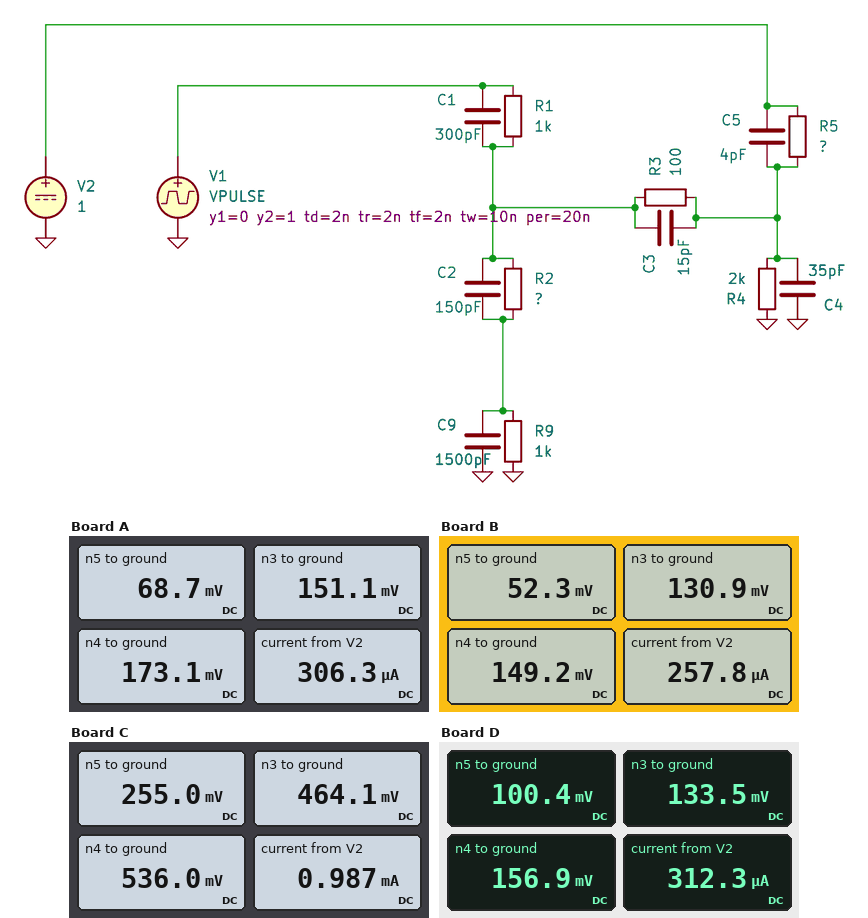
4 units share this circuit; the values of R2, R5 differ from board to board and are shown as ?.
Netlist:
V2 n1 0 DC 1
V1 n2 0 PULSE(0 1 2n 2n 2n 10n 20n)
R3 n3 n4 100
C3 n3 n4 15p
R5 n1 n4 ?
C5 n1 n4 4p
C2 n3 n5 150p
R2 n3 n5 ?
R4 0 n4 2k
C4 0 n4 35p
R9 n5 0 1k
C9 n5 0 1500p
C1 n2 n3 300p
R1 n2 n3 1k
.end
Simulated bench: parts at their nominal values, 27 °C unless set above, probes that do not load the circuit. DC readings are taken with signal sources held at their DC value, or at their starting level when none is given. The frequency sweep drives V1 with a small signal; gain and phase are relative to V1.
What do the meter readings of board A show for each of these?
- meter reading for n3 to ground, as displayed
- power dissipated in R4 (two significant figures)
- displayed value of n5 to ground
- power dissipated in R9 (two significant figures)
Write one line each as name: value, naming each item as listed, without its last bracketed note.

meter reading for n3 to ground, as displayed: 151.1 mV
power dissipated in R4: 15 µW
displayed value of n5 to ground: 68.7 mV
power dissipated in R9: 4.7 µW
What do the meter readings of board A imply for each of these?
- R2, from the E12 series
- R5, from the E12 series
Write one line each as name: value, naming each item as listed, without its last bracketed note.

R2, from the E12 series: 1.2 kΩ
R5, from the E12 series: 2.7 kΩ
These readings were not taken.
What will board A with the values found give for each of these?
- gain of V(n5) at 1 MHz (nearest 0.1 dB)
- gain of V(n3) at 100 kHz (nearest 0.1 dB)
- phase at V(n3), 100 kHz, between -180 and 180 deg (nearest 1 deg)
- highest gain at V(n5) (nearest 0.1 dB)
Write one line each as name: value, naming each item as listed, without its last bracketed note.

gain of V(n5) at 1 MHz: -23.7 dB
gain of V(n3) at 100 kHz: -7.3 dB
phase at V(n3), 100 kHz, between -180 and 180 deg: 1 deg
highest gain at V(n5): -13.9 dB
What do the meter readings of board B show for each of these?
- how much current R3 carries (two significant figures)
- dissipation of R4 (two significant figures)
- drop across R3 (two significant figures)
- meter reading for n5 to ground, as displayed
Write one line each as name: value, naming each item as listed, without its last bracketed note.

how much current R3 carries: 180 µA
dissipation of R4: 11 µW
drop across R3: 18 mV
meter reading for n5 to ground, as displayed: 52.3 mV
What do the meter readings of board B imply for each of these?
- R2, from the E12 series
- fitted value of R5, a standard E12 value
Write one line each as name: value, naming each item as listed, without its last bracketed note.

R2, from the E12 series: 1.5 kΩ
fitted value of R5, a standard E12 value: 3.3 kΩ
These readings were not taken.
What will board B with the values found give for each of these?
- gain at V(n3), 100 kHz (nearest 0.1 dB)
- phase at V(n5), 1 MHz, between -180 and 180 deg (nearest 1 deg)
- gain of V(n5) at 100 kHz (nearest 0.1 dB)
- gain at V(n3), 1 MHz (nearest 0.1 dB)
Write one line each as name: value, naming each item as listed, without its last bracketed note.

gain at V(n3), 100 kHz: -6.8 dB
phase at V(n5), 1 MHz, between -180 and 180 deg: -16 deg
gain of V(n5) at 100 kHz: -16.1 dB
gain at V(n3), 1 MHz: -4.9 dB
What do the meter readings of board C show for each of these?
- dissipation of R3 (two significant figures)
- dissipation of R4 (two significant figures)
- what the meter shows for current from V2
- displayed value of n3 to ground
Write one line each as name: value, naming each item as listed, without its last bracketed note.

dissipation of R3: 52 µW
dissipation of R4: 140 µW
what the meter shows for current from V2: 0.987 mA
displayed value of n3 to ground: 464.1 mV
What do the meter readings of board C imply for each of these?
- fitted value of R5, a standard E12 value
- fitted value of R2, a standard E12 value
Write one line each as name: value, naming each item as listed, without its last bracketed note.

fitted value of R5, a standard E12 value: 470 Ω
fitted value of R2, a standard E12 value: 820 Ω
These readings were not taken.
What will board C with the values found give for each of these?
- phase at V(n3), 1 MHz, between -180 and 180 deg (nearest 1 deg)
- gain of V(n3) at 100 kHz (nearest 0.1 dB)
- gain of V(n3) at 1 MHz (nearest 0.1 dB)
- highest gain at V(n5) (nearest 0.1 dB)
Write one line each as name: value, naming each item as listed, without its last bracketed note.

phase at V(n3), 1 MHz, between -180 and 180 deg: 26 deg
gain of V(n3) at 100 kHz: -11.3 dB
gain of V(n3) at 1 MHz: -7.5 dB
highest gain at V(n5): -16.4 dB
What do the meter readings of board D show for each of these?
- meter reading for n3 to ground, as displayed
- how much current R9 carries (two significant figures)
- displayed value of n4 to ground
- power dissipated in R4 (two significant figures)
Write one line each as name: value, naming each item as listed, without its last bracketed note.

meter reading for n3 to ground, as displayed: 133.5 mV
how much current R9 carries: 100 µA
displayed value of n4 to ground: 156.9 mV
power dissipated in R4: 12 µW
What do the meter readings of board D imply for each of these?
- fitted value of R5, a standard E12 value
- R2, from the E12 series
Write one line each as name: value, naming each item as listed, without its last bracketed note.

fitted value of R5, a standard E12 value: 2.7 kΩ
R2, from the E12 series: 330 Ω
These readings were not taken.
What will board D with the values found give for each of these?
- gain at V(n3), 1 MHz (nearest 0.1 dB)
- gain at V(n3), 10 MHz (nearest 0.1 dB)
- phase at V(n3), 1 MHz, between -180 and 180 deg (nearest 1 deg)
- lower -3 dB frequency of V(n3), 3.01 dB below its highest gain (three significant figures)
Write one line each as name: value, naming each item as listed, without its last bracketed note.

gain at V(n3), 1 MHz: -8.1 dB
gain at V(n3), 10 MHz: -4.0 dB
phase at V(n3), 1 MHz, between -180 and 180 deg: 21 deg
lower -3 dB frequency of V(n3), 3.01 dB below its highest gain: 1.56 MHz
